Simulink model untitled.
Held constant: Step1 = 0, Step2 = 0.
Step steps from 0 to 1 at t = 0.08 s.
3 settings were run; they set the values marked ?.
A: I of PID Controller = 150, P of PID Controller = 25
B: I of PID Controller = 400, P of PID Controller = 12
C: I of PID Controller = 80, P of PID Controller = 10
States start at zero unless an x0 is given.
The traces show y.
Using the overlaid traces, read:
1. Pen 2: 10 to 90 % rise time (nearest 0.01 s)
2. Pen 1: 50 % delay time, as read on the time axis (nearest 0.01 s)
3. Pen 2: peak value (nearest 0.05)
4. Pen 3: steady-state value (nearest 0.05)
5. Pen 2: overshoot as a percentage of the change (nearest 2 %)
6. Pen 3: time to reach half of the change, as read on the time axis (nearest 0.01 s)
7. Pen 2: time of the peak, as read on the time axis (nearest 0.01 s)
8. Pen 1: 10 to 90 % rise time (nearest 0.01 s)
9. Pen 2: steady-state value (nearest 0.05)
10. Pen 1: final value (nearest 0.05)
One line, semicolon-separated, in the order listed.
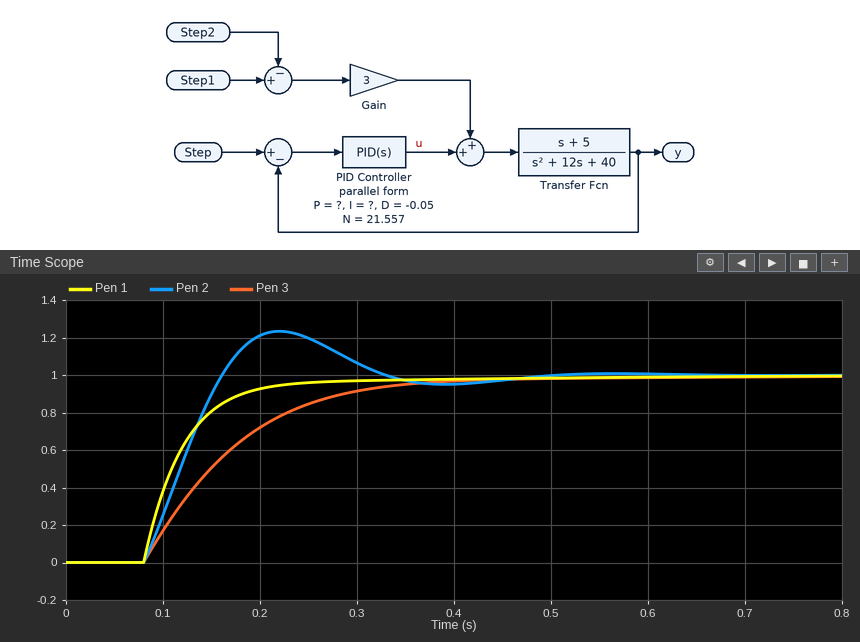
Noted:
0.06 s; 0.11 s; 1.25; 1.00; 24 %; 0.15 s; 0.22 s; 0.10 s; 1.00; 1.00
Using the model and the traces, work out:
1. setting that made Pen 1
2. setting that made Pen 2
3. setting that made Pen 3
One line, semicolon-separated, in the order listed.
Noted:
A; B; C
